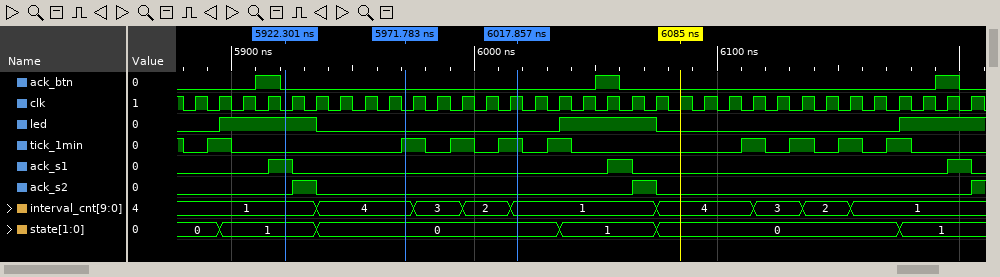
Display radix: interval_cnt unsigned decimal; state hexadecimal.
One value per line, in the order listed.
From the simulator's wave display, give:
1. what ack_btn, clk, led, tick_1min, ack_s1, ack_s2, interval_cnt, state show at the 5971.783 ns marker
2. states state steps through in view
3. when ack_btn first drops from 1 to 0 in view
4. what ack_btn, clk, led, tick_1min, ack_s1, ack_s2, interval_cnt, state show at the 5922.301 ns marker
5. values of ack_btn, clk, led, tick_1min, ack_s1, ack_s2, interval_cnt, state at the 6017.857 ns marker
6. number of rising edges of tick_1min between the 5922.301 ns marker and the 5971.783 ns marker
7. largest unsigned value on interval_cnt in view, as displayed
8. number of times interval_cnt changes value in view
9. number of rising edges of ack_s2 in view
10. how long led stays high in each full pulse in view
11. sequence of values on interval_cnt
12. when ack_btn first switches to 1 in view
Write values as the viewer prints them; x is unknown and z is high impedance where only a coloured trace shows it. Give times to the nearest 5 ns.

ack_btn=0, clk=0, led=0, tick_1min=1, ack_s1=0, ack_s2=0, interval_cnt=4, state=0
0, 1, 0, 1, 0, 1
5920 ns
ack_btn=0, clk=0, led=1, tick_1min=0, ack_s1=1, ack_s2=0, interval_cnt=1, state=1
ack_btn=0, clk=1, led=0, tick_1min=1, ack_s1=0, ack_s2=0, interval_cnt=1, state=0
1
4
8
3
40 ns, 40 ns
1, 4, 3, 2, 1, 4, 3, 2, 1
5910 ns
